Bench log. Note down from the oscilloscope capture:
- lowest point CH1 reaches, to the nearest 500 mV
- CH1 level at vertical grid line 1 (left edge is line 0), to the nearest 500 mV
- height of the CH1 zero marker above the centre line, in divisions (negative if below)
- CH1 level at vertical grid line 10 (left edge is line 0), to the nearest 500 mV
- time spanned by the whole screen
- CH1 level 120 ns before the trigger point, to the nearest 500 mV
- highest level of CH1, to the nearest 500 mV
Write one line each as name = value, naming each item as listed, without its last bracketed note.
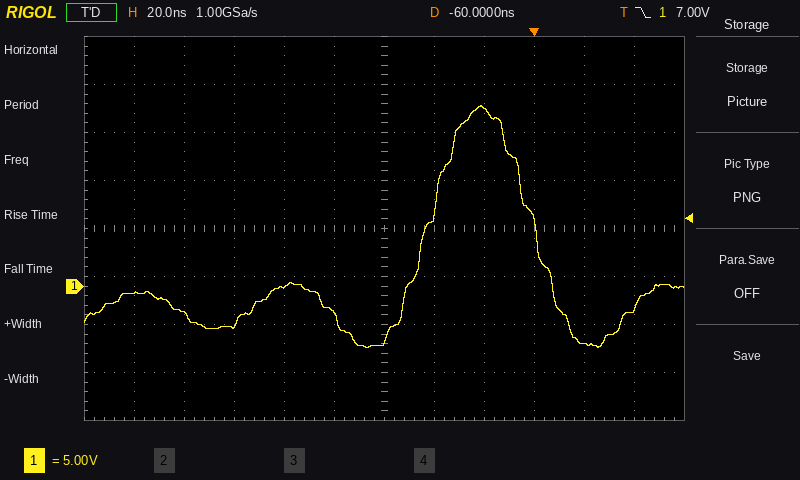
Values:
lowest point CH1 reaches, to the nearest 500 mV = -6.5 V
CH1 level at vertical grid line 1 (left edge is line 0), to the nearest 500 mV = -500 mV
height of the CH1 zero marker above the centre line, in divisions = -1.2 div
CH1 level at vertical grid line 10 (left edge is line 0), to the nearest 500 mV = -6.0 V
time spanned by the whole screen = 240 ns
CH1 level 120 ns before the trigger point, to the nearest 500 mV = -4.0 V
highest level of CH1, to the nearest 500 mV = 19.0 V
